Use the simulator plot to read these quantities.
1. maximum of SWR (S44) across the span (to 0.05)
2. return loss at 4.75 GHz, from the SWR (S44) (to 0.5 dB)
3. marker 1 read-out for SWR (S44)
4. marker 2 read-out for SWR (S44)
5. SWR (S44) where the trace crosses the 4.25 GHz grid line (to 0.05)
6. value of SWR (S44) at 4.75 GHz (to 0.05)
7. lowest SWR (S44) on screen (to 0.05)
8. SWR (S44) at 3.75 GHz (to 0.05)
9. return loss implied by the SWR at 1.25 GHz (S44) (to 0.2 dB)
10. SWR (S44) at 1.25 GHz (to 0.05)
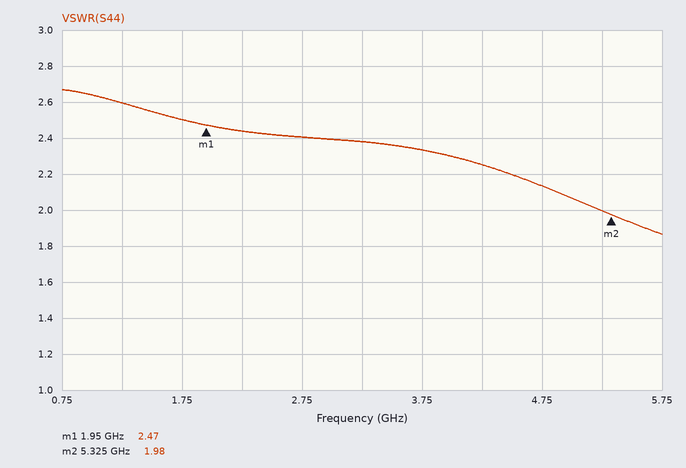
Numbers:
2.65
9.0 dB
2.47
1.98
2.25
2.15
1.85
2.35
7.0 dB
2.60
